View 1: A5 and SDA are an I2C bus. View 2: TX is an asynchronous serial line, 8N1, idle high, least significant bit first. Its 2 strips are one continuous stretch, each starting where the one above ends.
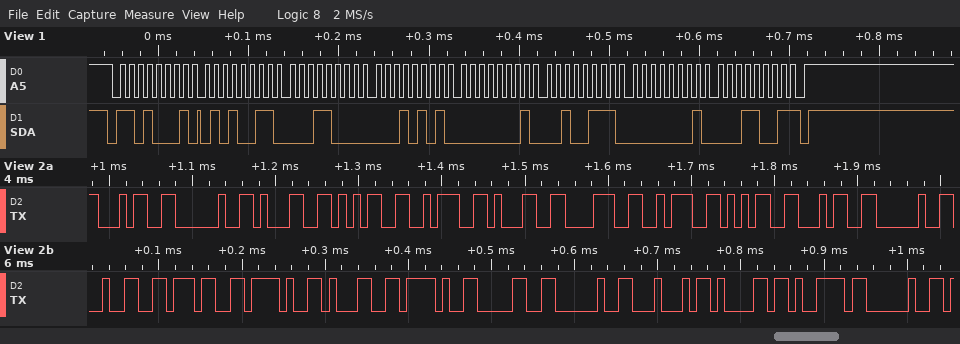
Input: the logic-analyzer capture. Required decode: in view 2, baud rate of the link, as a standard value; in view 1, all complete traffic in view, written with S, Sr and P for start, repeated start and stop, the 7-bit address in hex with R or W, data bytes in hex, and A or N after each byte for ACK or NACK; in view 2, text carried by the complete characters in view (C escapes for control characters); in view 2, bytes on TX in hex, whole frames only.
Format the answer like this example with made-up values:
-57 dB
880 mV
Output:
115200 baud
S 68R A 53 A 18 A 15 A 01 A 27 A 01 A 19 N P
"4 15:18:54 27/1/0 Day "
34 20 31 35 3A 31 38 3A 35 34 20 32 37 2F 31 2F 30 20 44 61 79 20
